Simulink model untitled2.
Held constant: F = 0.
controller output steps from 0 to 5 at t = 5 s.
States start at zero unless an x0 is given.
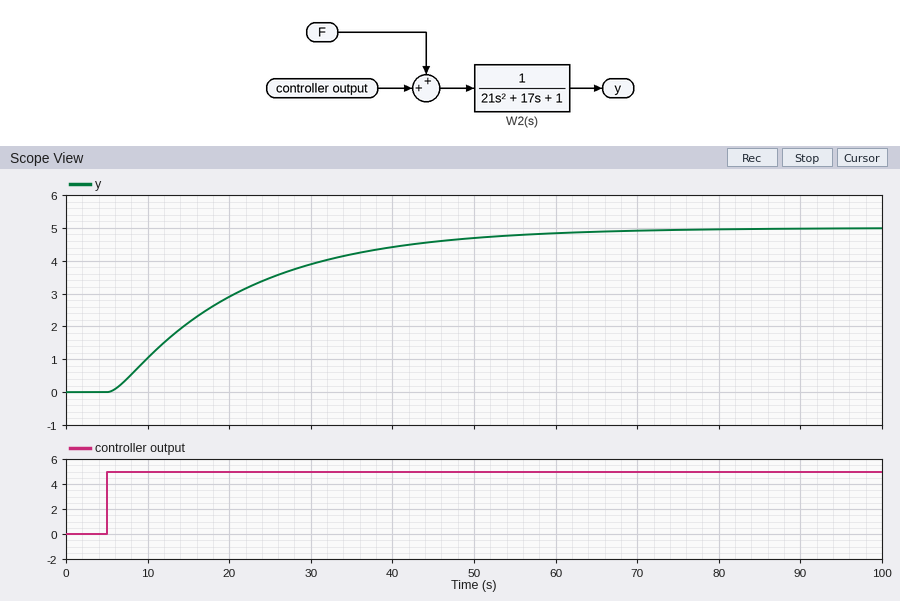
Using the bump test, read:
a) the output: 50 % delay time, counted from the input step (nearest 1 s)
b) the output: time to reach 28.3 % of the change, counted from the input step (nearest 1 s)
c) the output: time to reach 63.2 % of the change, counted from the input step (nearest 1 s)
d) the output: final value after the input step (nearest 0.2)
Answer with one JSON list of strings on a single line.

["12 s", "7 s", "17 s", "5.0"]
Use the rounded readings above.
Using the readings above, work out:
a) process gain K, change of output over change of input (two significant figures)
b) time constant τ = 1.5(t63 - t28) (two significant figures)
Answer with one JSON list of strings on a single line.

["1.0", "15 s"]
